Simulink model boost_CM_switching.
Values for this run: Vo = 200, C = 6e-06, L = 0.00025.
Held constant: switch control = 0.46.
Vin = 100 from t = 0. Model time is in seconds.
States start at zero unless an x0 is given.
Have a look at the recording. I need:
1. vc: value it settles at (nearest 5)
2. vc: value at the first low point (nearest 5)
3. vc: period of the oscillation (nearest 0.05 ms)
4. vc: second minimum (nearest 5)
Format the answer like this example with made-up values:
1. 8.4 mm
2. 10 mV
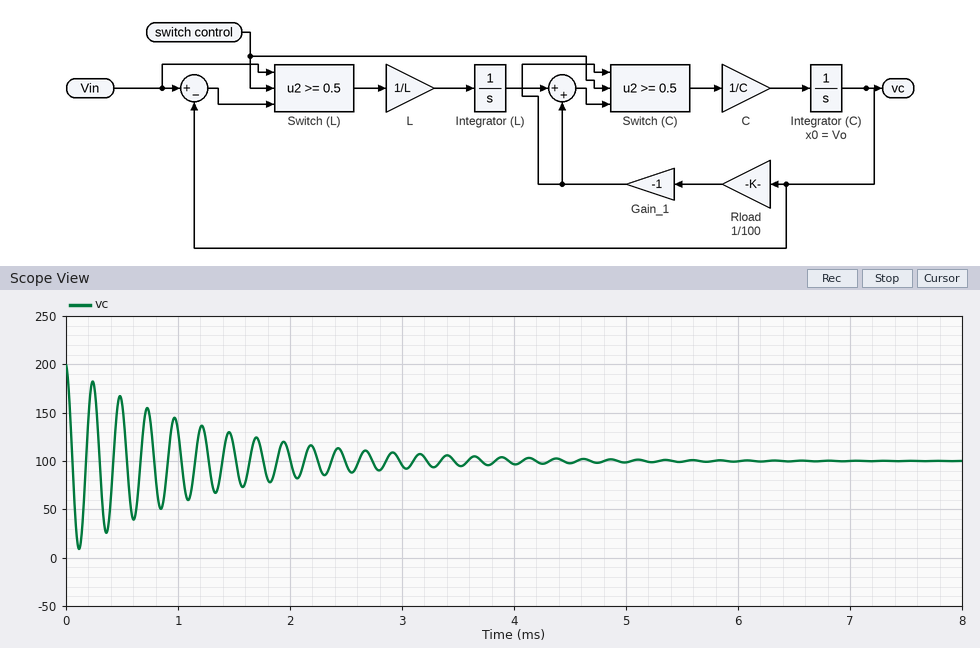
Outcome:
1. 100
2. 10
3. 0.25 ms
4. 25
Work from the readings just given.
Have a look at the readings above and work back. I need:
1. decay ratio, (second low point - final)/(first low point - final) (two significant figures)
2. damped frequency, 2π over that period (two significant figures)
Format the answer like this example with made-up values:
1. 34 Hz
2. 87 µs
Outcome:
1. 0.83
2. 25 rad/ms
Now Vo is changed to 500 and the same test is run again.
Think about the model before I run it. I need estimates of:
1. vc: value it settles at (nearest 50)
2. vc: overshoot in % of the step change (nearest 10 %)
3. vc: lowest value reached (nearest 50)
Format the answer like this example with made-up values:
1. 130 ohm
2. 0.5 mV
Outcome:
1. 100
2. 90 %
3. -250
